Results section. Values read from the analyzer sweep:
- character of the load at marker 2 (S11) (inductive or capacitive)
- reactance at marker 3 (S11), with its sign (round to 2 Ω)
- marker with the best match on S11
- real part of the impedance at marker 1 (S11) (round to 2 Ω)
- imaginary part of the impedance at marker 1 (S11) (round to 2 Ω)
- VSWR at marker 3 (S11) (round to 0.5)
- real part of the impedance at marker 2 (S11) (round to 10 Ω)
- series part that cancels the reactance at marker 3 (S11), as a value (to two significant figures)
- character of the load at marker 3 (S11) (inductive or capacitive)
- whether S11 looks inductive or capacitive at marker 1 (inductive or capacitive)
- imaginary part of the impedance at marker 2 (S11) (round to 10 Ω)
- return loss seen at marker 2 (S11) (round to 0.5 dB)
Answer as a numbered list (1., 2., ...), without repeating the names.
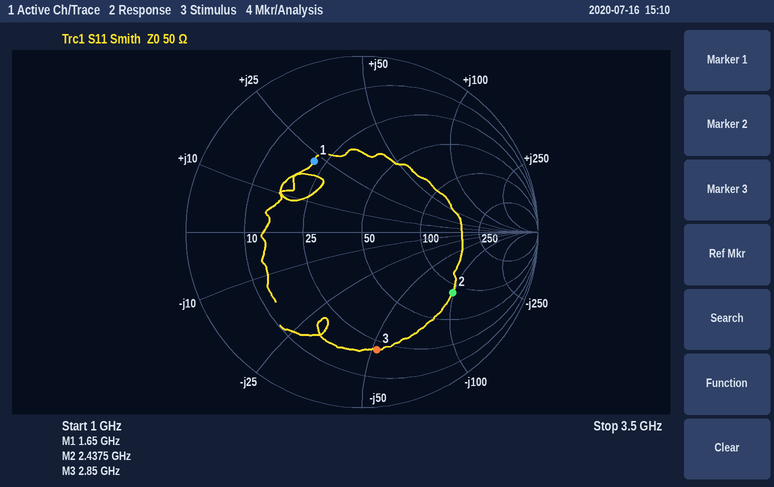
1. capacitive
2. -52 Ω
3. marker 1
4. 22 Ω
5. +22 Ω
6. 5.0
7. 90 Ω
8. 2.9 nH
9. capacitive
10. inductive
11. -100 Ω
12. 4.0 dB
